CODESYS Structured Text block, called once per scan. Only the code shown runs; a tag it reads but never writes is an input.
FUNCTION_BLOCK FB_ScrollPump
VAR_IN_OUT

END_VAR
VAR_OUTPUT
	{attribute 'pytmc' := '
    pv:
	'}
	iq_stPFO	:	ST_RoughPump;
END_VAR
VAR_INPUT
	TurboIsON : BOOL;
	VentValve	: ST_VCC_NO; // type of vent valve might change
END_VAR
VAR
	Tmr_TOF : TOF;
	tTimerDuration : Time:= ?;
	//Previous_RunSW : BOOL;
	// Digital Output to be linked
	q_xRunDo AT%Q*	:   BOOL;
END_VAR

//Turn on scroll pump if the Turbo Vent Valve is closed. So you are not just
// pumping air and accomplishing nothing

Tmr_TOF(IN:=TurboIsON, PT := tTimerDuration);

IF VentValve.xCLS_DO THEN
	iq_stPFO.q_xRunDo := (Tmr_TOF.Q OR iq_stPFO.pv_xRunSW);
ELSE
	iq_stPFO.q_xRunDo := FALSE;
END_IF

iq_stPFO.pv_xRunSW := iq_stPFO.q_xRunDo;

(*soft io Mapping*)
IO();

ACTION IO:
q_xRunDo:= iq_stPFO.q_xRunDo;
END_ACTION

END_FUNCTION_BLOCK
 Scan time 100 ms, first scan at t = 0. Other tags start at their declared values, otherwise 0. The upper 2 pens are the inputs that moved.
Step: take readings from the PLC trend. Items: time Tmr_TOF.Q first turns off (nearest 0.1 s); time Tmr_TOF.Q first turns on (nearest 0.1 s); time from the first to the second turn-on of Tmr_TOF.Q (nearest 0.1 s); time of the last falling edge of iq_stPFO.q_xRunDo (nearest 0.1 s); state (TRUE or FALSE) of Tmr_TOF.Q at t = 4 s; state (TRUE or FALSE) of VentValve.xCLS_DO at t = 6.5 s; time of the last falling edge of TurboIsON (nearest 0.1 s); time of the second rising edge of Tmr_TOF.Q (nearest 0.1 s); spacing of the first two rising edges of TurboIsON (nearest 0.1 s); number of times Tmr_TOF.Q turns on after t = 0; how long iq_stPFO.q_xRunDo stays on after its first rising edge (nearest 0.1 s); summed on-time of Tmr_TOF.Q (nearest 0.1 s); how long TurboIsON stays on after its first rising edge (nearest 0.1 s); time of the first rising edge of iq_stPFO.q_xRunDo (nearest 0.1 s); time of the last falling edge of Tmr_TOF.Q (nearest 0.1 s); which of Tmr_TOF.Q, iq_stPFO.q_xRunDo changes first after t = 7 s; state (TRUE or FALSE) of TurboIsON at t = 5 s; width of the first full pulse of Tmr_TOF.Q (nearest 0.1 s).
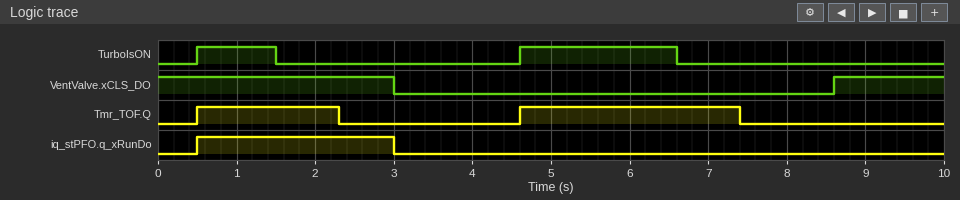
2.3 s
0.5 s
4.1 s
3.0 s
FALSE
FALSE
6.6 s
4.6 s
4.1 s
2
2.5 s
4.6 s
1.0 s
0.5 s
7.4 s
Tmr_TOF.Q
TRUE
1.8 s
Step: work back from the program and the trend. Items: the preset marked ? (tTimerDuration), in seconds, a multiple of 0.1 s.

0.8 s
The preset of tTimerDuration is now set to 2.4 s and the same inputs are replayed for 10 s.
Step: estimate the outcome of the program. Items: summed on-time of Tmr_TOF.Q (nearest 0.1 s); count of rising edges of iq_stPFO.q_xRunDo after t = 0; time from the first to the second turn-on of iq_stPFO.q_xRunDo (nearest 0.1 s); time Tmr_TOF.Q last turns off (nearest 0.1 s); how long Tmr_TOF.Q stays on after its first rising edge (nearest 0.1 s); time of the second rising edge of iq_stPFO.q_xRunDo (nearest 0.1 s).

7.8 s
2
8.1 s
9.0 s
3.4 s
8.6 s
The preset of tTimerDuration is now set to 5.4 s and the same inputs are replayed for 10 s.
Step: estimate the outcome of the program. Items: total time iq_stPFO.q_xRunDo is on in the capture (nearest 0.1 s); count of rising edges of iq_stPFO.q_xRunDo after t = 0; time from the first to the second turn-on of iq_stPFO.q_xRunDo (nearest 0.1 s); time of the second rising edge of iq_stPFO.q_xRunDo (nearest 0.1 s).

3.9 s
2
8.1 s
8.6 s
